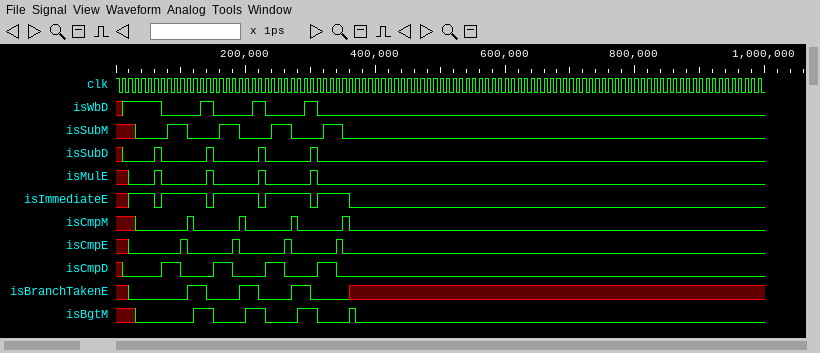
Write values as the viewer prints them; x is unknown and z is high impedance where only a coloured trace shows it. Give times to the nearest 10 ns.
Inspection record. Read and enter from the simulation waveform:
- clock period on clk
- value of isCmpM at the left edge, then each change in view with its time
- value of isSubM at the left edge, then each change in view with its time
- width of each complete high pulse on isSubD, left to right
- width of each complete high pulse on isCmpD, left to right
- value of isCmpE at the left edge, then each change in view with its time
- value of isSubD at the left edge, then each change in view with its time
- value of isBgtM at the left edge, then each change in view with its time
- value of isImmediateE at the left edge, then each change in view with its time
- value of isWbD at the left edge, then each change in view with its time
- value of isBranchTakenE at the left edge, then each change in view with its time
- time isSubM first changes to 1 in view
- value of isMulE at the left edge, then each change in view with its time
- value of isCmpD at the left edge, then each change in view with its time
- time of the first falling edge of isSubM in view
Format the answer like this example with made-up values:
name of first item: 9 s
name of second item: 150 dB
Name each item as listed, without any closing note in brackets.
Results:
clock period on clk: 10 ns
value of isCmpM at the left edge, then each change in view with its time: x, 0 at 30 ns, 1 at 110 ns, 0 at 120 ns, 1 at 190 ns, 0 at 200 ns, 1 at 270 ns, 0 at 280 ns, 1 at 350 ns, 0 at 360 ns
value of isSubM at the left edge, then each change in view with its time: x, 0 at 30 ns, 1 at 80 ns, 0 at 110 ns, 1 at 160 ns, 0 at 190 ns, 1 at 240 ns, 0 at 270 ns, 1 at 320 ns, 0 at 350 ns
width of each complete high pulse on isSubD, left to right: 10 ns, 10 ns, 10 ns, 10 ns
width of each complete high pulse on isCmpD, left to right: 30 ns, 30 ns, 30 ns, 30 ns
value of isCmpE at the left edge, then each change in view with its time: x, 0 at 20 ns, 1 at 100 ns, 0 at 110 ns, 1 at 180 ns, 0 at 190 ns, 1 at 260 ns, 0 at 270 ns, 1 at 340 ns, 0 at 350 ns
value of isSubD at the left edge, then each change in view with its time: x, 0 at 10 ns, 1 at 60 ns, 0 at 70 ns, 1 at 140 ns, 0 at 150 ns, 1 at 220 ns, 0 at 230 ns, 1 at 300 ns, 0 at 310 ns
value of isBgtM at the left edge, then each change in view with its time: x, 0 at 30 ns, 1 at 120 ns, 0 at 150 ns, 1 at 200 ns, 0 at 230 ns, 1 at 280 ns, 0 at 310 ns, 1 at 360 ns, 0 at 370 ns
value of isImmediateE at the left edge, then each change in view with its time: x, 1 at 20 ns, 0 at 60 ns, 1 at 70 ns, 0 at 140 ns, 1 at 150 ns, 0 at 220 ns, 1 at 230 ns, 0 at 300 ns, 1 at 310 ns, 0 at 360 ns
value of isWbD at the left edge, then each change in view with its time: x, 1 at 10 ns, 0 at 70 ns, 1 at 130 ns, 0 at 150 ns, 1 at 210 ns, 0 at 230 ns, 1 at 290 ns, 0 at 310 ns
value of isBranchTakenE at the left edge, then each change in view with its time: x, 0 at 20 ns, 1 at 110 ns, 0 at 140 ns, 1 at 190 ns, 0 at 220 ns, 1 at 270 ns, 0 at 300 ns, x at 360 ns
time isSubM first changes to 1 in view: 80 ns
value of isMulE at the left edge, then each change in view with its time: x, 0 at 20 ns, 1 at 60 ns, 0 at 70 ns, 1 at 140 ns, 0 at 150 ns, 1 at 220 ns, 0 at 230 ns, 1 at 300 ns, 0 at 310 ns
value of isCmpD at the left edge, then each change in view with its time: x, 0 at 10 ns, 1 at 70 ns, 0 at 100 ns, 1 at 150 ns, 0 at 180 ns, 1 at 230 ns, 0 at 260 ns, 1 at 310 ns, 0 at 340 ns
time of the first falling edge of isSubM in view: 110 ns
